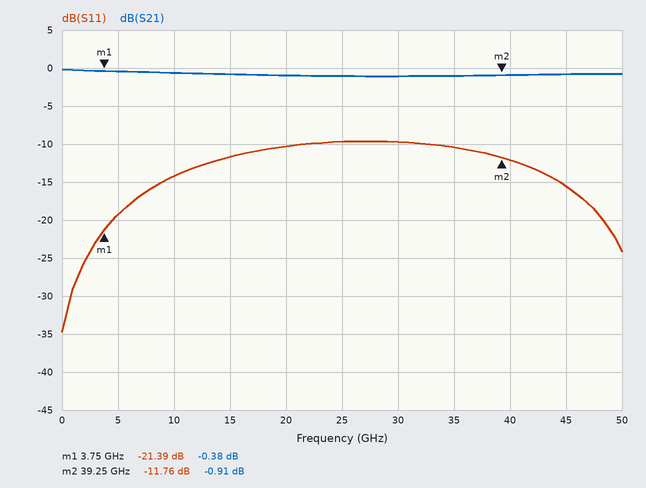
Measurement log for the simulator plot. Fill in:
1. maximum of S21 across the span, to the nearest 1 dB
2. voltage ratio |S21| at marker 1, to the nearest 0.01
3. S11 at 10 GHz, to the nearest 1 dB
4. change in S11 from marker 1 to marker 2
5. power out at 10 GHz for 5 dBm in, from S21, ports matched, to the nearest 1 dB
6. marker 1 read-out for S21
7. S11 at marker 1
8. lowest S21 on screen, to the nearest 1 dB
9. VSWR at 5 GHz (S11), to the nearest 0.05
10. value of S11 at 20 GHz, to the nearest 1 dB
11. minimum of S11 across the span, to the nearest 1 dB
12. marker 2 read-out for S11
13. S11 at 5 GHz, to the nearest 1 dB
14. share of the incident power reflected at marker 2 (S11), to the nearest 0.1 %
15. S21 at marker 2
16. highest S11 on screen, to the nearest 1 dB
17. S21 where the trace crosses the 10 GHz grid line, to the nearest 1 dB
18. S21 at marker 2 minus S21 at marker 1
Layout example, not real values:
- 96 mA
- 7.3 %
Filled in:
- 0 dB
- 0.96
- -14 dB
- 9.63 dB
- 4 dBm
- -0.38 dB
- -21.39 dB
- -1 dB
- 1.25
- -10 dB
- -35 dB
- -11.76 dB
- -19 dB
- 6.7 %
- -0.91 dB
- -10 dB
- -1 dB
- -0.53 dB
